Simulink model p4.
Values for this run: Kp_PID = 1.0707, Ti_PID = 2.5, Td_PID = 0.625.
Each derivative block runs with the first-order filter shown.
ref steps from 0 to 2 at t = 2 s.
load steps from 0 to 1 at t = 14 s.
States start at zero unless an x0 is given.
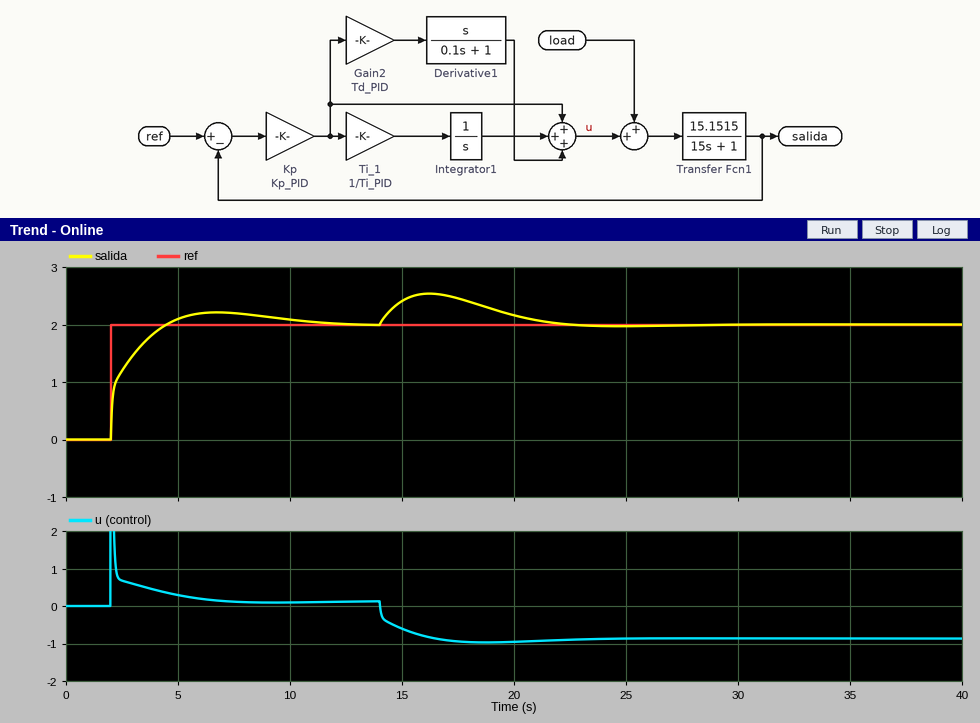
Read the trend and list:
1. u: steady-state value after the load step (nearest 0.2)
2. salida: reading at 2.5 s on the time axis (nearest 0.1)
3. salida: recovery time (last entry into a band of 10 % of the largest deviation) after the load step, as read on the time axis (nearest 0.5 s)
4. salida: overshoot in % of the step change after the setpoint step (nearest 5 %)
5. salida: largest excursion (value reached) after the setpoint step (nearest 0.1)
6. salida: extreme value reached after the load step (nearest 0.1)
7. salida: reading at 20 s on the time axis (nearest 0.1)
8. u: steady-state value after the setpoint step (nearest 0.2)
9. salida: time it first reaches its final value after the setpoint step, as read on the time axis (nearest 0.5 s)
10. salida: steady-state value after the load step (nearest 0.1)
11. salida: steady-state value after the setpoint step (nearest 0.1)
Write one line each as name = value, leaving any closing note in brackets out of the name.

u: steady-state value after the load step = -0.8
salida: reading at 2.5 s on the time axis = 1.2
salida: recovery time (last entry into a band of 10 % of the largest deviation) after the load step, as read on the time axis = 21.5 s
salida: overshoot in % of the step change after the setpoint step = 10 %
salida: largest excursion (value reached) after the setpoint step = 2.2
salida: extreme value reached after the load step = 2.5
salida: reading at 20 s on the time axis = 2.2
u: steady-state value after the setpoint step = 0.2
salida: time it first reaches its final value after the setpoint step, as read on the time axis = 4.5 s
salida: steady-state value after the load step = 2.0
salida: steady-state value after the setpoint step = 2.0
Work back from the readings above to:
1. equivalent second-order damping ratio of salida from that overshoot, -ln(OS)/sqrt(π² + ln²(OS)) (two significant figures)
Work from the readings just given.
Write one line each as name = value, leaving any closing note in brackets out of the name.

equivalent second-order damping ratio of salida from that overshoot, -ln(OS)/sqrt(π² + ln²(OS)) = 0.59
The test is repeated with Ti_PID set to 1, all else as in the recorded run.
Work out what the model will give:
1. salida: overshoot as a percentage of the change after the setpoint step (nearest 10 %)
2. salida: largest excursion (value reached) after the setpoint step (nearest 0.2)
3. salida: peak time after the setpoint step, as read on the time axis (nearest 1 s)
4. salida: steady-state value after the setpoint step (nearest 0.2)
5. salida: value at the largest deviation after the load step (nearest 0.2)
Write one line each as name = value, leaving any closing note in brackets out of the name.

salida: overshoot as a percentage of the change after the setpoint step = 20 %
salida: largest excursion (value reached) after the setpoint step = 2.4
salida: peak time after the setpoint step, as read on the time axis = 5 s
salida: steady-state value after the setpoint step = 2.0
salida: value at the largest deviation after the load step = 2.4
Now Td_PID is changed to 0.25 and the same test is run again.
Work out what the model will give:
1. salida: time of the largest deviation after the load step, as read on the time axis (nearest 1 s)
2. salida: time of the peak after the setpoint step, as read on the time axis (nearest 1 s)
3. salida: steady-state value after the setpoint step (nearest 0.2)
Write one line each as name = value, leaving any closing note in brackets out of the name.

salida: time of the largest deviation after the load step, as read on the time axis = 16 s
salida: time of the peak after the setpoint step, as read on the time axis = 6 s
salida: steady-state value after the setpoint step = 2.0
